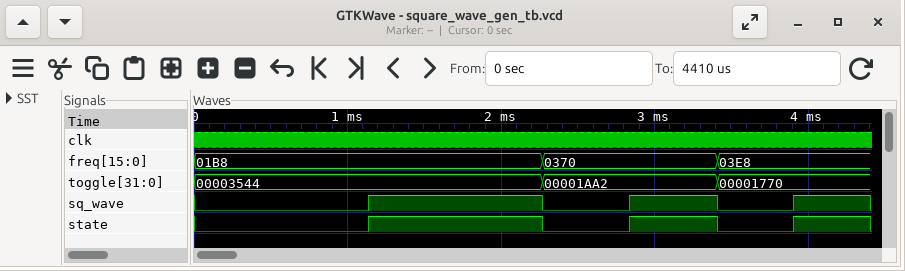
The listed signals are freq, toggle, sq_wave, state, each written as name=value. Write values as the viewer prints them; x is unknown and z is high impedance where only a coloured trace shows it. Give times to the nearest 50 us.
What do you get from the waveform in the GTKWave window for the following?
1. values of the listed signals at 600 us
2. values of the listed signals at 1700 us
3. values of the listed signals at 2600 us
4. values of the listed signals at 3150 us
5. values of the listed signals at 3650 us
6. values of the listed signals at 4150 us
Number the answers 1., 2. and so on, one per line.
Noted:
1. freq=01B8, toggle=00003544, sq_wave=0, state=0
2. freq=01B8, toggle=00003544, sq_wave=1, state=1
3. freq=0370, toggle=00001AA2, sq_wave=0, state=0
4. freq=0370, toggle=00001AA2, sq_wave=1, state=1
5. freq=03E8, toggle=00001770, sq_wave=0, state=0
6. freq=03E8, toggle=00001770, sq_wave=1, state=1
